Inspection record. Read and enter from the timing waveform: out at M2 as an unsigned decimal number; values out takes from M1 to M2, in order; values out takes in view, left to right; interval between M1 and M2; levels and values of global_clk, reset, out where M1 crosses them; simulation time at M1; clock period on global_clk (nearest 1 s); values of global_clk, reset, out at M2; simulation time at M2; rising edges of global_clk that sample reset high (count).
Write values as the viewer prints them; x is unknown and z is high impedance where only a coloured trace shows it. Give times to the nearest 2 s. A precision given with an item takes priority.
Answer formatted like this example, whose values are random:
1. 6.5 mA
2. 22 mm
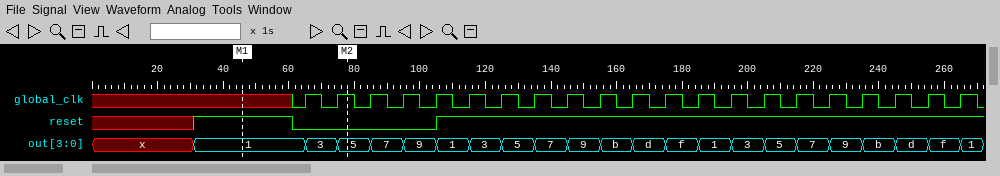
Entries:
1. 5
2. 1, 3, 5
3. x, 1, 3, 5, 7, 9, 1, 3, 5, 7, 9, b, d, f, 1, 3, 5, 7, 9, b, d, f, 1
4. 32 s
5. global_clk=x, reset=1, out=1
6. 46 s
7. 10 s
8. global_clk=1, reset=0, out=5
9. 78 s
10. 16
